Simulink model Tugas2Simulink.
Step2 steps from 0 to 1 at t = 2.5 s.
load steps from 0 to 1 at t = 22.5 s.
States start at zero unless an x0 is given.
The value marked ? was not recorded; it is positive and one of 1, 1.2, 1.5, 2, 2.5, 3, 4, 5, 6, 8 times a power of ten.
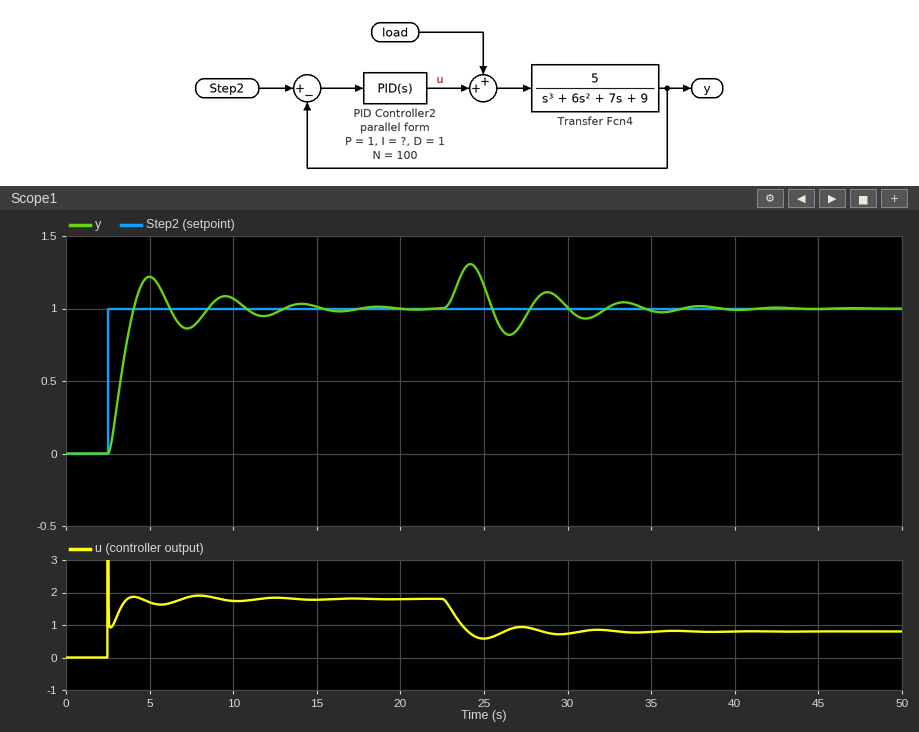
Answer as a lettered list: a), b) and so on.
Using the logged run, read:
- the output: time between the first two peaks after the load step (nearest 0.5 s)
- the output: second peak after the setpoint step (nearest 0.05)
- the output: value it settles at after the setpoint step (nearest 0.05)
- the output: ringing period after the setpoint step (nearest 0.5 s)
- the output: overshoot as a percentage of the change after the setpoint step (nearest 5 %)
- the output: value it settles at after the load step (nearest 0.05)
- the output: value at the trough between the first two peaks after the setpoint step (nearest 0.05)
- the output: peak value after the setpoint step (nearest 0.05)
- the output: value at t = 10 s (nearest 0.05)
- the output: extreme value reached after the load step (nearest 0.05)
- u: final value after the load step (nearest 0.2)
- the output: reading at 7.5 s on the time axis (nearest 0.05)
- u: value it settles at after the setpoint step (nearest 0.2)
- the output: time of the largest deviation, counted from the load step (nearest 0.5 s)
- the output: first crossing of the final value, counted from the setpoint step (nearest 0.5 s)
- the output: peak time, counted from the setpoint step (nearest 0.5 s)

a) 4.5 s
b) 1.10
c) 1.00
d) 4.5 s
e) 20 %
f) 1.00
g) 0.85
h) 1.20
i) 1.05
j) 1.30
k) 0.8
l) 0.85
m) 1.8
n) 1.5 s
o) 1.5 s
p) 2.5 s
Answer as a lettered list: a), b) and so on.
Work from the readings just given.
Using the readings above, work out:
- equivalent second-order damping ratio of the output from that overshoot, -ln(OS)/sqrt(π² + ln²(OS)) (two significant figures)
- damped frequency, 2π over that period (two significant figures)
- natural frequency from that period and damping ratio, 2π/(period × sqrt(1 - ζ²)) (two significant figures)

a) 0.46
b) 1.4 rad/s
c) 1.6 rad/s
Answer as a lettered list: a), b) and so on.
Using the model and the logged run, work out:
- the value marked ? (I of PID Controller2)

a) 3
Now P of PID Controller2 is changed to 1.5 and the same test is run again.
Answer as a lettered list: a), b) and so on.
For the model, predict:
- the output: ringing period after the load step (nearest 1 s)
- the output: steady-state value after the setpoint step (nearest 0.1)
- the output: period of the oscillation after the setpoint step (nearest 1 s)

a) 4 s
b) 1.0
c) 4 s
